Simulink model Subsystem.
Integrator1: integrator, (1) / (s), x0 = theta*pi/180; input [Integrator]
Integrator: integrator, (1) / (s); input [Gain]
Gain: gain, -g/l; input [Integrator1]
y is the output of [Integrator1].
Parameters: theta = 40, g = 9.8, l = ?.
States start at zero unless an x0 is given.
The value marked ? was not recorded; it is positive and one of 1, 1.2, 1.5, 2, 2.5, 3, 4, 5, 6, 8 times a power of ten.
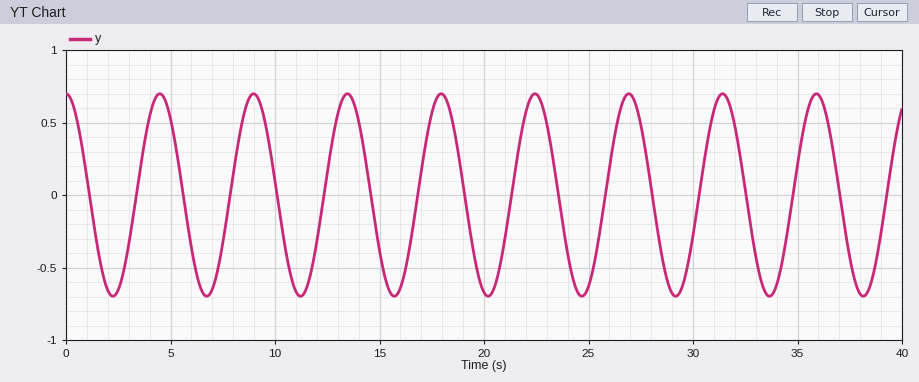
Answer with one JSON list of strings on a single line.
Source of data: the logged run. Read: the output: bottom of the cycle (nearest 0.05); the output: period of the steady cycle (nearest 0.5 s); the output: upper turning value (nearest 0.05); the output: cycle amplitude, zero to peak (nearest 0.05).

["-0.70", "4.5 s", "0.70", "0.70"]
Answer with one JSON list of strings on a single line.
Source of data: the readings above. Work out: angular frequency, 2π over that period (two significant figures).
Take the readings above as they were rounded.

["1.4 rad/s"]
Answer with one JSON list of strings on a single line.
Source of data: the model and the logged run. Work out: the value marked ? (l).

["5"]
